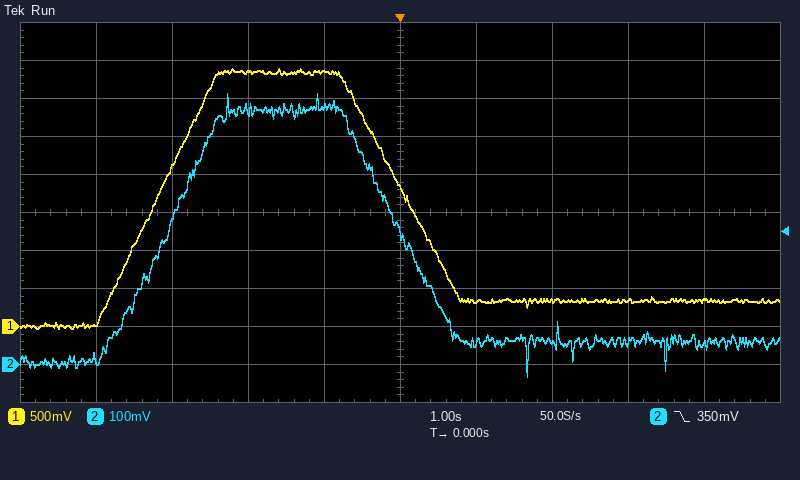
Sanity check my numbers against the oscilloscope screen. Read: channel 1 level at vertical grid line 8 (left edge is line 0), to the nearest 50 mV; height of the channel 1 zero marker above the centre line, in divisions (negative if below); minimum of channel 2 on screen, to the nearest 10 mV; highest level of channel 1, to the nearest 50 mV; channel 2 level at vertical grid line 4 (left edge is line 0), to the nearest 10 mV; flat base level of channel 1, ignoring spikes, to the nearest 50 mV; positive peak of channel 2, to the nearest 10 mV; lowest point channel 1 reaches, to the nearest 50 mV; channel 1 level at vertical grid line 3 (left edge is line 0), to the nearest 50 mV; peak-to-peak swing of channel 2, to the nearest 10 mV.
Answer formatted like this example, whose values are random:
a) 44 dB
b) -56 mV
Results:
a) 350 mV
b) -3.0 div
c) -30 mV
d) 3.40 V
e) 680 mV
f) 350 mV
g) 710 mV
h) -50 mV
i) 3.35 V
j) 740 mV
